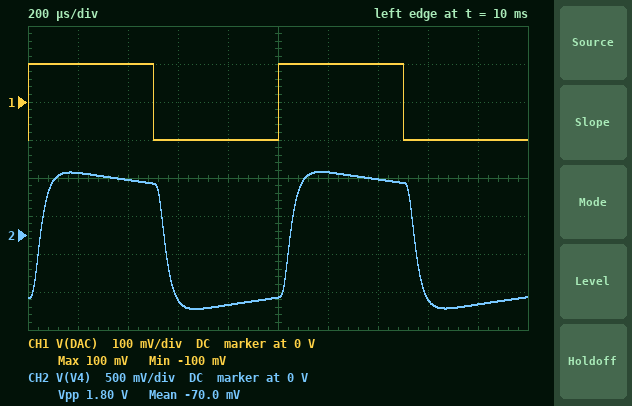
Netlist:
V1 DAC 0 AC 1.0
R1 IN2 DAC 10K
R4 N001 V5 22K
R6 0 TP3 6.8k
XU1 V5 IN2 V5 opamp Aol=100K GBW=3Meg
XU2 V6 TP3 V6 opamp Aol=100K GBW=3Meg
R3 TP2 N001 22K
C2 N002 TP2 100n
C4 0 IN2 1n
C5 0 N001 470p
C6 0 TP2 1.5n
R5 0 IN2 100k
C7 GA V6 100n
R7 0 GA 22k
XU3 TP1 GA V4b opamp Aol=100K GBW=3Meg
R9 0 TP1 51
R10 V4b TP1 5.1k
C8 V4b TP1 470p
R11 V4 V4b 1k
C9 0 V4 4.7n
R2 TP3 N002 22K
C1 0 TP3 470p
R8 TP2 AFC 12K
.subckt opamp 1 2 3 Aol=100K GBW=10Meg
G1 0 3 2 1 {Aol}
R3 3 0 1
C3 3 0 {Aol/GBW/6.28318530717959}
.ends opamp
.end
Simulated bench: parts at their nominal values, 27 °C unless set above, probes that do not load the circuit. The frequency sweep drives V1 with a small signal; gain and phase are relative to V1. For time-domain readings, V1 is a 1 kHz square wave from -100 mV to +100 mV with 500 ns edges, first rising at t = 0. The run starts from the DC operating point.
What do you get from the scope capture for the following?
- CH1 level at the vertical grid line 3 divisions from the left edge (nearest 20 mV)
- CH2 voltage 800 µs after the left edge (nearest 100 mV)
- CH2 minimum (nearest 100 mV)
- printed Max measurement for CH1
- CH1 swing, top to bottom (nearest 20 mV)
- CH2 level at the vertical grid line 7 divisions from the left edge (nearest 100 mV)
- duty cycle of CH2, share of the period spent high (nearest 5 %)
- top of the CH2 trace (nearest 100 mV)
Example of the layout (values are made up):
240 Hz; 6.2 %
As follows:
-100 mV; -900 mV; -1.0 V; 100 mV; 200 mV; 700 mV; 50 %; 800 mV
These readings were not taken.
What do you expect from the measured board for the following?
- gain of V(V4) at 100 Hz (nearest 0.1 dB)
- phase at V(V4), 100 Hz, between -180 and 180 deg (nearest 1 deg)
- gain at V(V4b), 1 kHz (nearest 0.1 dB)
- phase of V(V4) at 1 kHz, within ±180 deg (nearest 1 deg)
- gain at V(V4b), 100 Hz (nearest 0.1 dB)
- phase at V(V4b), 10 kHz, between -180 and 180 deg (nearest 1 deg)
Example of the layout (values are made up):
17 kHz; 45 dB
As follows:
16.6 dB; 46 deg; 18.4 dB; -15 deg; 16.6 dB; -142 deg
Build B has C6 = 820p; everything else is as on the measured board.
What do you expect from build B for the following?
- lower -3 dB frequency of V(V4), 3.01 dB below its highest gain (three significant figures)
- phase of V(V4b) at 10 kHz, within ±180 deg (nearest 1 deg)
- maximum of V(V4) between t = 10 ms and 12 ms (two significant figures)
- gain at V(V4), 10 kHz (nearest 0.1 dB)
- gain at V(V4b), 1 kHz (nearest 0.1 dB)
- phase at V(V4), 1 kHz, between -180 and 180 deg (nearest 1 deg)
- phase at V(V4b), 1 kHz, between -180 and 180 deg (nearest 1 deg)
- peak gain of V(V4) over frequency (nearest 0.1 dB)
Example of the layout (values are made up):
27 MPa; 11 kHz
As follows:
76.7 Hz; -127 deg; 850 mV; 12.2 dB; 18.5 dB; -11 deg; -9 deg; 18.5 dB
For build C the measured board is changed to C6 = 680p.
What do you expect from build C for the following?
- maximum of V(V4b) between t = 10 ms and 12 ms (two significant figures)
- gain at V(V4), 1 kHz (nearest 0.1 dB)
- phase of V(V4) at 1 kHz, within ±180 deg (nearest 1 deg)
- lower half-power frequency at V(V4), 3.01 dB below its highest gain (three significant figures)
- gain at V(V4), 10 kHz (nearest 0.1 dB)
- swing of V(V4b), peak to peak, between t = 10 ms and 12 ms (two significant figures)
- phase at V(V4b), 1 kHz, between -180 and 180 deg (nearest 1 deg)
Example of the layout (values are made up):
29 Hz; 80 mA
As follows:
860 mV; 18.5 dB; -10 deg; 76.8 Hz; 12.9 dB; 1.9 V; -9 deg
